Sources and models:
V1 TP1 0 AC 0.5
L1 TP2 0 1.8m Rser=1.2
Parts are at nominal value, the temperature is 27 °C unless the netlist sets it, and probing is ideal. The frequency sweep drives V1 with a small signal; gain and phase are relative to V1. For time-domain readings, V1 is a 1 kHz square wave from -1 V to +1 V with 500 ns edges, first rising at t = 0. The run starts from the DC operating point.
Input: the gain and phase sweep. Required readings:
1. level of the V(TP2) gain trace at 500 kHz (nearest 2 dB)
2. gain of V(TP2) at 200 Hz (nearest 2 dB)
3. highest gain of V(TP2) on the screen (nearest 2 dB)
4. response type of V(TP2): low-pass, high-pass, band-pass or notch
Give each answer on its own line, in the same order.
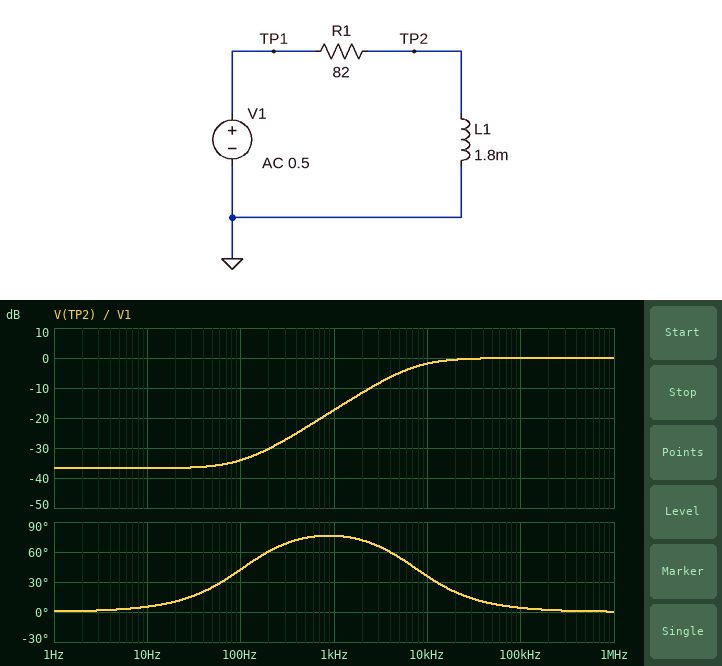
0 dB
-30 dB
0 dB
high-pass
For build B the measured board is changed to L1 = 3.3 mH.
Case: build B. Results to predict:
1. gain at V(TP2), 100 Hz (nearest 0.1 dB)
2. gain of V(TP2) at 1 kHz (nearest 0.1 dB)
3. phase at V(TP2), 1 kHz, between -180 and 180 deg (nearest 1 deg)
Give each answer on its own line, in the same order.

-30.8 dB
-12.3 dB
73 deg
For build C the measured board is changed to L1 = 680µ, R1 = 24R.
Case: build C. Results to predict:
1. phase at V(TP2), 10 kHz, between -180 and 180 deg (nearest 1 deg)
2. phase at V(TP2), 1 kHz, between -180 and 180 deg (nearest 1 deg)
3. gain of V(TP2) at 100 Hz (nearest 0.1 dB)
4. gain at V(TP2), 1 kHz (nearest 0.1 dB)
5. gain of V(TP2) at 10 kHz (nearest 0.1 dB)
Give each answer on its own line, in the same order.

29 deg
65 deg
-25.9 dB
-15.2 dB
-1.3 dB
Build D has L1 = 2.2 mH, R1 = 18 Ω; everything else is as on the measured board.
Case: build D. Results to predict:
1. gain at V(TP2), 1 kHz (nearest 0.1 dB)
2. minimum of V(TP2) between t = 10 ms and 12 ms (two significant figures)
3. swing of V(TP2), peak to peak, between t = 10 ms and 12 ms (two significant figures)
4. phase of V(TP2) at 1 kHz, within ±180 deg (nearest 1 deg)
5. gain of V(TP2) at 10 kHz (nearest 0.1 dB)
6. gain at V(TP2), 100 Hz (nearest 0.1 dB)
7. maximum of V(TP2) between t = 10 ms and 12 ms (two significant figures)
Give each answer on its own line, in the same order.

-4.6 dB
-1.9 V
3.8 V
49 deg
-0.1 dB
-20.4 dB
1.9 V
